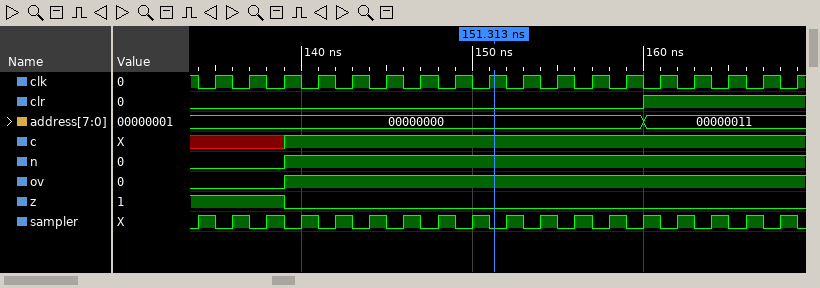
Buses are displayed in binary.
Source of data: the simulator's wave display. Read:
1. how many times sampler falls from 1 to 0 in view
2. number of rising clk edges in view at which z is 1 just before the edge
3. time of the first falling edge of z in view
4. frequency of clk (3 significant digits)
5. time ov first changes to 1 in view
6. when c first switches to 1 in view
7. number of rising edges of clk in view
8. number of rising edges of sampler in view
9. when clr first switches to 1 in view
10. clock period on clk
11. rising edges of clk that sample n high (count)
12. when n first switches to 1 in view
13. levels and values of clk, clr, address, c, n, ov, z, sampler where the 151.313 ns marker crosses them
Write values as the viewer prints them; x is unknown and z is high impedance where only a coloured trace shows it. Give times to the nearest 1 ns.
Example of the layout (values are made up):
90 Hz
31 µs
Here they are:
18
3
139 ns
500 MHz
139 ns
139 ns
18
18
160 ns
2 ns
15
139 ns
clk=1, clr=0, address=00000000, c=1, n=1, ov=1, z=0, sampler=0
